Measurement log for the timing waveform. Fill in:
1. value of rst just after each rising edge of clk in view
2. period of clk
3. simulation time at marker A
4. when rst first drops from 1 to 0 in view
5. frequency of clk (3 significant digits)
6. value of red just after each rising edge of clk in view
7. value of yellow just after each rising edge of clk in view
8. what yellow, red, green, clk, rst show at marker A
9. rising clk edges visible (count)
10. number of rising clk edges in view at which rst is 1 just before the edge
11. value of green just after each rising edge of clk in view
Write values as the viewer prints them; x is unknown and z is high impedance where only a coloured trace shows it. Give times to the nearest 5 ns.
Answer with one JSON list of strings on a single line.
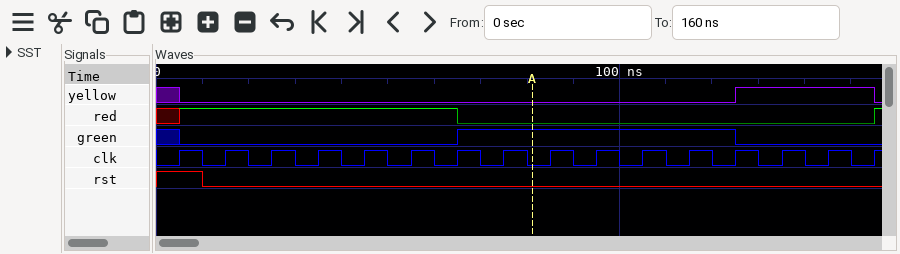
["1 0 0 0 0 0 0 0 0 0 0 0 0 0 0 0", "10 ns", "80 ns", "10 ns", "100 MHz", "1 1 1 1 1 1 0 0 0 0 0 0 0 0 0 1", "0 0 0 0 0 0 0 0 0 0 0 0 1 1 1 0", "yellow=0, red=0, green=1, clk=0, rst=0", "16", "1", "0 0 0 0 0 0 1 1 1 1 1 1 0 0 0 0"]
